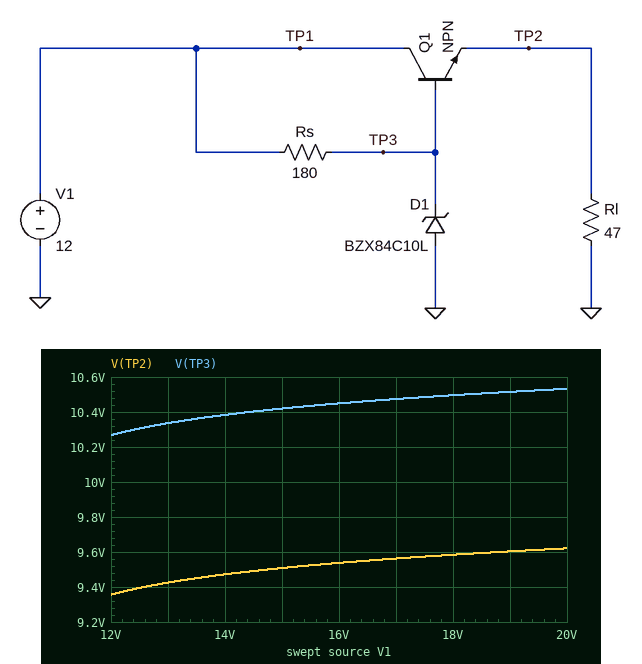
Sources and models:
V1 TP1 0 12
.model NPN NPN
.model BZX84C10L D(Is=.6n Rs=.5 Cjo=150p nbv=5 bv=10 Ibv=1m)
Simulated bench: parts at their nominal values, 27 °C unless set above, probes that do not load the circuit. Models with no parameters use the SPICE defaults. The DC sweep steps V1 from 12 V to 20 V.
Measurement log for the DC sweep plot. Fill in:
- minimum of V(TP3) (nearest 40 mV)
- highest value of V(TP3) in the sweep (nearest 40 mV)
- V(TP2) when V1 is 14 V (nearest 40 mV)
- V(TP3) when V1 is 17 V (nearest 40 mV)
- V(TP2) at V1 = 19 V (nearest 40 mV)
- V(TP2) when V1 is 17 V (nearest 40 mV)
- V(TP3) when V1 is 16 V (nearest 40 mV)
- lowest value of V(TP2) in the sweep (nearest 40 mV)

10.28 V
10.52 V
9.48 V
10.48 V
9.60 V
9.56 V
10.44 V
9.36 V
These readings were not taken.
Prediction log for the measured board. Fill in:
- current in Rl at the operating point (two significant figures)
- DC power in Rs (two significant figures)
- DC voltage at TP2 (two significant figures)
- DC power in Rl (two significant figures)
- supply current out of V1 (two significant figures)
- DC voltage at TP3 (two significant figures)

200 mA
17 mW
9.4 V
1.9 W
210 mA
10 V
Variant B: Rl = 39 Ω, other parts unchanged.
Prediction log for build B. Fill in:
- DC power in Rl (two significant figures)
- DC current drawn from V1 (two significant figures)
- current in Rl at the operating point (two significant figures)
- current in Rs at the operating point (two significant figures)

2.2 W
250 mA
240 mA
9.7 mA
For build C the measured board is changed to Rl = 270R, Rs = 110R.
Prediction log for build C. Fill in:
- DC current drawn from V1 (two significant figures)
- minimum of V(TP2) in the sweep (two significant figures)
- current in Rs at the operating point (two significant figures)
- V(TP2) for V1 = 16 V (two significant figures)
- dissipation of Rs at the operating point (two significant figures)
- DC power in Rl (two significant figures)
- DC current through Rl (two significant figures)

50 mA
9.5 V
15 mA
9.7 V
25 mW
330 mW
35 mA
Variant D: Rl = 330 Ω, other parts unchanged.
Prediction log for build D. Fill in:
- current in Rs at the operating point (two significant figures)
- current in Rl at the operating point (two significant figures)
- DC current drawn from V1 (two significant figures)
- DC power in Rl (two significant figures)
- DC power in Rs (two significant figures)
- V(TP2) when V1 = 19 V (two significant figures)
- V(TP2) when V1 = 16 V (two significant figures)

9.5 mA
29 mA
38 mA
270 mW
16 mW
9.7 V
9.6 V
